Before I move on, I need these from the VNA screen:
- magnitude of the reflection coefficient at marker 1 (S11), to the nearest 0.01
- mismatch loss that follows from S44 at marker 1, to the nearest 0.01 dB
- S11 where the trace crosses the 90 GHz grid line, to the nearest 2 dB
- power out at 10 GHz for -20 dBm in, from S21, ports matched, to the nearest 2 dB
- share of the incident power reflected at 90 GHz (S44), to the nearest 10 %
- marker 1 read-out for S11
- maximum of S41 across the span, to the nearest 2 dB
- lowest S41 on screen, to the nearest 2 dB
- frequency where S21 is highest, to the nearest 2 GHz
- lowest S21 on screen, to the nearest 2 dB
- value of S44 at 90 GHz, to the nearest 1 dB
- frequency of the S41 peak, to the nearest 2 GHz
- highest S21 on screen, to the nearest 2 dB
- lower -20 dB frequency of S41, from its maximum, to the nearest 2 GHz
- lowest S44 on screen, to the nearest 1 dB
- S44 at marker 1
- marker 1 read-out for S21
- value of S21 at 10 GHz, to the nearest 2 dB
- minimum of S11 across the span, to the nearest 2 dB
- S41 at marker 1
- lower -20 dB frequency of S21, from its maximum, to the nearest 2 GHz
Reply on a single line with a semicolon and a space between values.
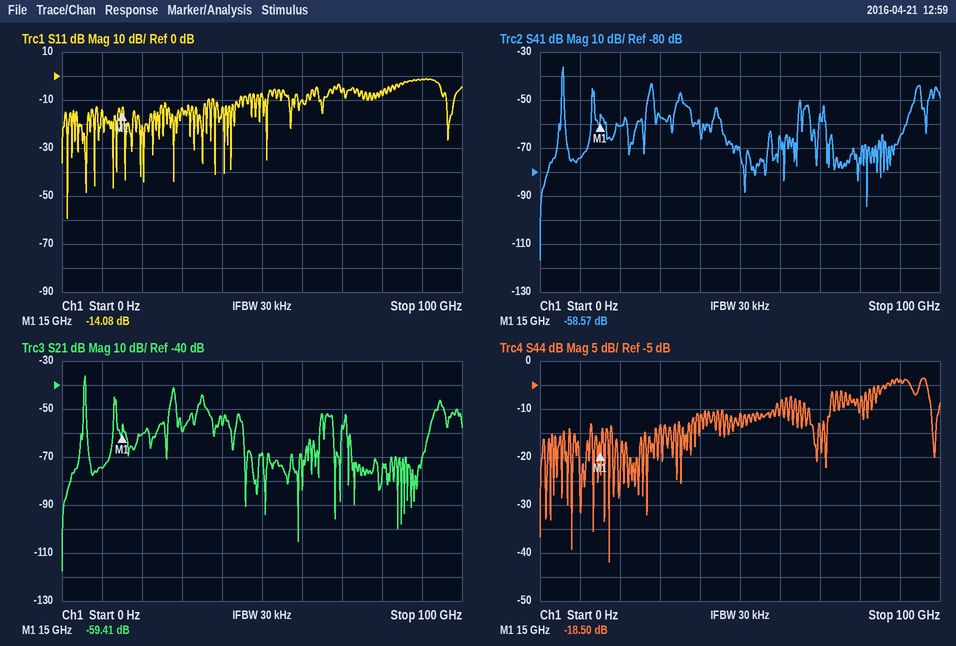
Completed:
0.20; 0.06 dB; -2 dB; -94 dBm; 40 %; -14.08 dB; -36 dB; -116 dB; 6 GHz; -118 dB; -4 dB; 6 GHz; -36 dB; 6 GHz; -42 dB; -18.50 dB; -59.41 dB; -74 dB; -60 dB; -58.57 dB; 6 GHz
